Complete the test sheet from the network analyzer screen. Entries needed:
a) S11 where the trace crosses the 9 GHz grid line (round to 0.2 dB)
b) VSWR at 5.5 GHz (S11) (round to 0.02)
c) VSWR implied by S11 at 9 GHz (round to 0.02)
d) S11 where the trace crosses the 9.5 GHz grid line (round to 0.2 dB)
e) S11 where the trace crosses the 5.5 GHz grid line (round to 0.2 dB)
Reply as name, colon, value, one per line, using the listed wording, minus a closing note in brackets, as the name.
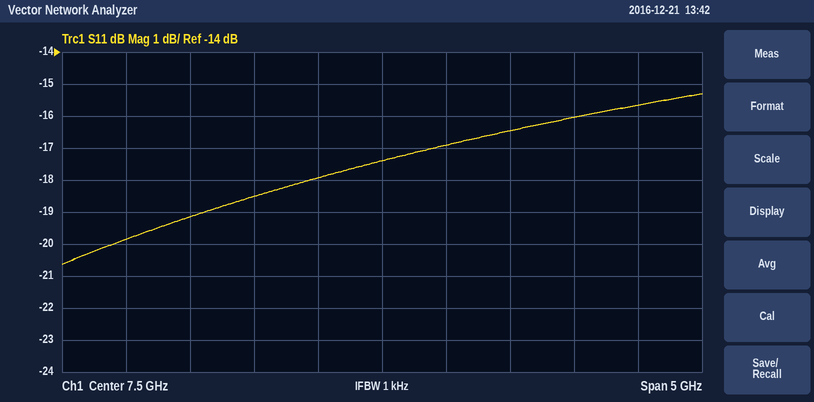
S11 where the trace crosses the 9 GHz grid line: -16.0 dB
VSWR at 5.5 GHz (S11): 1.22
VSWR implied by S11 at 9 GHz: 1.38
S11 where the trace crosses the 9.5 GHz grid line: -15.6 dB
S11 where the trace crosses the 5.5 GHz grid line: -19.8 dB
